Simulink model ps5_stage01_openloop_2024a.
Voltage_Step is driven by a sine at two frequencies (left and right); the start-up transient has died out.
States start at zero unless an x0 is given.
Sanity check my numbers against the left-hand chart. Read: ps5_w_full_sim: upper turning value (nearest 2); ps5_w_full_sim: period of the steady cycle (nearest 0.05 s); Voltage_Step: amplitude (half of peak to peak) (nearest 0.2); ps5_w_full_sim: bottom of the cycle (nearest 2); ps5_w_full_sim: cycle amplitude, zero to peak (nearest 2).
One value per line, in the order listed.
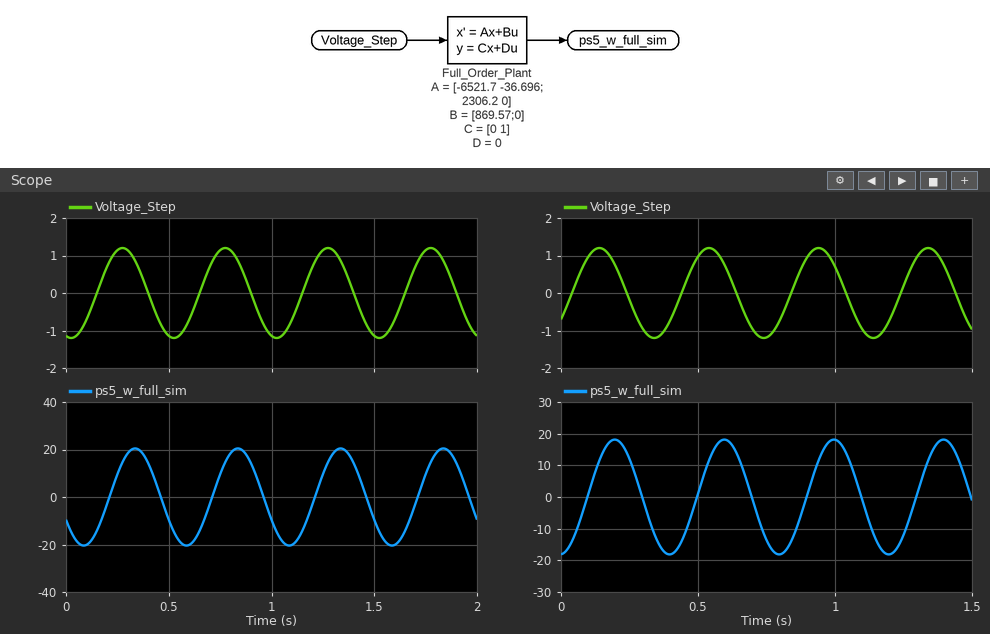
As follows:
20
0.50 s
1.2
-20
20
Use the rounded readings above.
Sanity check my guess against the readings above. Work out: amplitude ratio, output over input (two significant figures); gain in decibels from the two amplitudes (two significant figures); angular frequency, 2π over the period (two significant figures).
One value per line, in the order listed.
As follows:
17
24 dB
13 rad/s
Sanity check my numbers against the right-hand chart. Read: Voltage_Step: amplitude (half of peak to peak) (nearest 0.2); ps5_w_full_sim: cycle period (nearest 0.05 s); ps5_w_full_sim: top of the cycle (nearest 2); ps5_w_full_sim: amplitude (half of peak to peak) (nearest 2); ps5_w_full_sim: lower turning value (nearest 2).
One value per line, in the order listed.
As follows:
1.2
0.40 s
18
18
-18
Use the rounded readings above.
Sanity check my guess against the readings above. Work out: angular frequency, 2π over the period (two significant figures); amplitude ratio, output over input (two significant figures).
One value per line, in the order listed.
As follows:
16 rad/s
15
